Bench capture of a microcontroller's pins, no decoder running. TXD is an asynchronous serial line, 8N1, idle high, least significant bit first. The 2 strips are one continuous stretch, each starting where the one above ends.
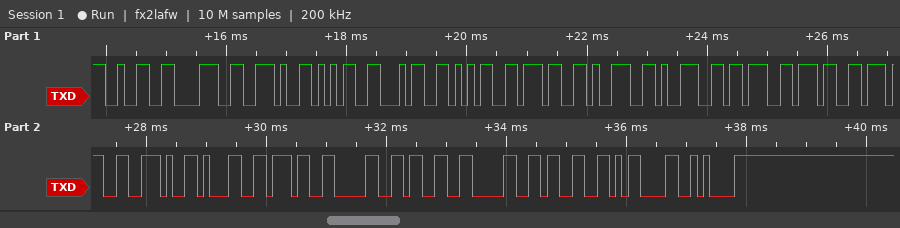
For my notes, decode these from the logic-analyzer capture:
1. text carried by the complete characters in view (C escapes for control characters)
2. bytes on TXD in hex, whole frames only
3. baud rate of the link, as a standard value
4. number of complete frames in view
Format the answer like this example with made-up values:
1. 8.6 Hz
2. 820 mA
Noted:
1. "28.545799;77.170303\r\n"
2. 32 38 2E 35 34 35 37 39 39 3B 37 37 2E 31 37 30 33 30 33 0D 0A
3. 9600 baud
4. 21
